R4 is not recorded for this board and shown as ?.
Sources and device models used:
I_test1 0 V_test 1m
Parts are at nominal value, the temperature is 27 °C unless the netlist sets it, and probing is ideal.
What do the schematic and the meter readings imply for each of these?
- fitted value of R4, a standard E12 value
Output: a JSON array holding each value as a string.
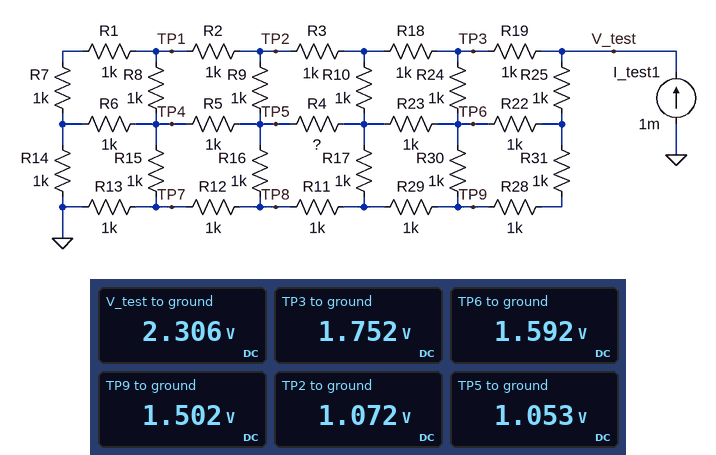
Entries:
["470 Ω"]
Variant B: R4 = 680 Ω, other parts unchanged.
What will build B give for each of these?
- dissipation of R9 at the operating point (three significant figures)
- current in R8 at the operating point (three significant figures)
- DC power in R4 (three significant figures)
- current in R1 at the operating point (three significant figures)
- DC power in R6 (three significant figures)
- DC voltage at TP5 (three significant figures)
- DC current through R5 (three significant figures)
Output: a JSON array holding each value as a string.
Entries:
["1.36 µW", "93.3 µA", "98.4 µW", "180 µA", "70.7 µW", "1.04 V", "329 µA"]
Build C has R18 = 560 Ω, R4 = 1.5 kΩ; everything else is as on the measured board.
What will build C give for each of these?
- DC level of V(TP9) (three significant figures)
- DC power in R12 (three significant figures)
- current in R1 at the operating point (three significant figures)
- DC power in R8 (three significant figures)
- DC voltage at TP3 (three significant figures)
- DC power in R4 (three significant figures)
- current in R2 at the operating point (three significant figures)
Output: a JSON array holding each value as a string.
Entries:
["1.57 V", "163 µW", "184 µA", "11.6 µW", "1.76 V", "102 µW", "292 µA"]
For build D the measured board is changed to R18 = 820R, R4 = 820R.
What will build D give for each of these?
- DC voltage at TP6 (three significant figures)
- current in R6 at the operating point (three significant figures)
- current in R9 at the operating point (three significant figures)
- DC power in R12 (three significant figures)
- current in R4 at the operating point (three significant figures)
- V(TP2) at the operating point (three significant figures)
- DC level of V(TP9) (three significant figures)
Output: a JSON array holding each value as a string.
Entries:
["1.63 V", "265 µA", "52.4 µA", "159 µW", "351 µA", "1.09 V", "1.54 V"]
